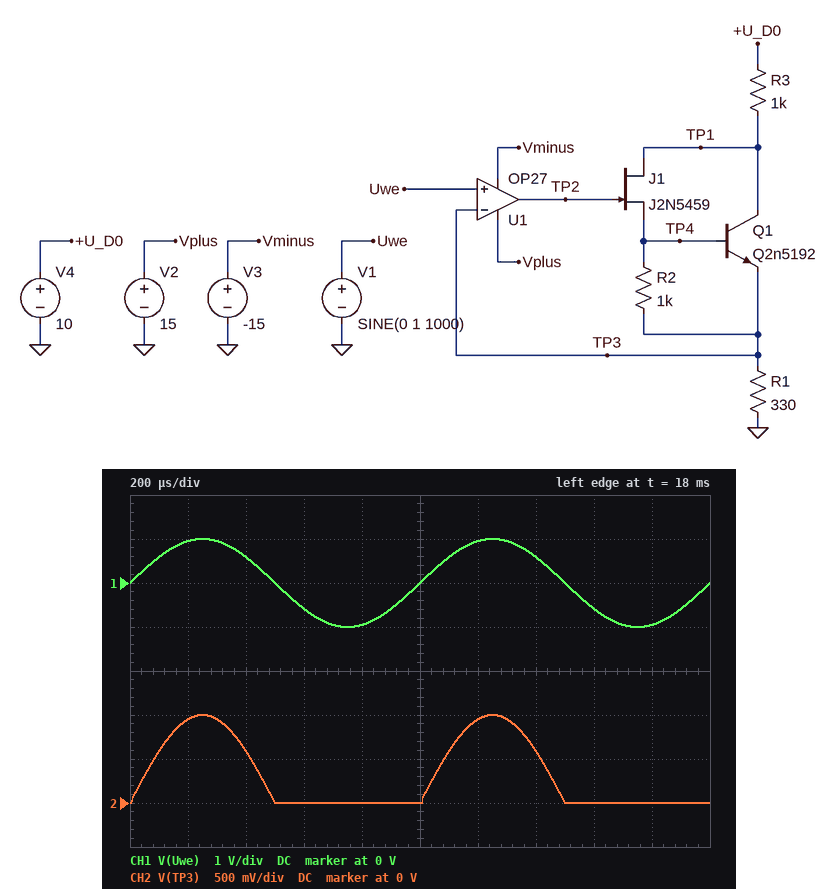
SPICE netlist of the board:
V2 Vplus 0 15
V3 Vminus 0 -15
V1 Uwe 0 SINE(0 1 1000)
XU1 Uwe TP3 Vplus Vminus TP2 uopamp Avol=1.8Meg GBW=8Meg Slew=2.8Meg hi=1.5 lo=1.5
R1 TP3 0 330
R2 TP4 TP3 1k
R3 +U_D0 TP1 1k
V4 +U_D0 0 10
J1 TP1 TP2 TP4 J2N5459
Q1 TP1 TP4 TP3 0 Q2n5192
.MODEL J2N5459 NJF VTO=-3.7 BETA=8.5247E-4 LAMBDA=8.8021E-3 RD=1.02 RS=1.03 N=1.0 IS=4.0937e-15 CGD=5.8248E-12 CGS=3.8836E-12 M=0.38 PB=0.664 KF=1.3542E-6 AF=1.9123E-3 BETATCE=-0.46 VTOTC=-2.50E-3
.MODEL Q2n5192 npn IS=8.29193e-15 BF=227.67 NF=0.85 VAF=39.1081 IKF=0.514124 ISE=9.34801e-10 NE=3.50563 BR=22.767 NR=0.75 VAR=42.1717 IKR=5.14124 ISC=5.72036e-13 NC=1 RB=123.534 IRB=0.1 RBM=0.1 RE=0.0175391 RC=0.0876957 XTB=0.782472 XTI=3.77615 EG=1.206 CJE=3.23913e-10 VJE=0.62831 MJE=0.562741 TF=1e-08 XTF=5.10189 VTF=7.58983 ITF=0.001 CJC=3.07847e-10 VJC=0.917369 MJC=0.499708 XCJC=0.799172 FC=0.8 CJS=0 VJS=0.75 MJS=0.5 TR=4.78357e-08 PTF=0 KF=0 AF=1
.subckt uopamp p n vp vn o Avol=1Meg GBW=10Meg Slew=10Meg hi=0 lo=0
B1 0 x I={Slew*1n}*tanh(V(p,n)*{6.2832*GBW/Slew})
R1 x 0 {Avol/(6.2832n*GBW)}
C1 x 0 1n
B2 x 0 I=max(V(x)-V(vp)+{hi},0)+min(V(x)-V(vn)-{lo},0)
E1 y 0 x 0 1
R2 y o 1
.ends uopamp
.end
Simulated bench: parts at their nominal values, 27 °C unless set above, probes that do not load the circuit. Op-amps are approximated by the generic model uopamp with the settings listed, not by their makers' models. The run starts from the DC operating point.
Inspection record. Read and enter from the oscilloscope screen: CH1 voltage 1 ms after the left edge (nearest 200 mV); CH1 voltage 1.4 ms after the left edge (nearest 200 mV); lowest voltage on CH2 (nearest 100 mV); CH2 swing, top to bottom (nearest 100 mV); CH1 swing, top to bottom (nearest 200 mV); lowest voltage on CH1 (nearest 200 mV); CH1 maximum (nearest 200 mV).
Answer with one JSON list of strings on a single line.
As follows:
["0 V", "600 mV", "0 V", "1.0 V", "2.0 V", "-1.0 V", "1.0 V"]
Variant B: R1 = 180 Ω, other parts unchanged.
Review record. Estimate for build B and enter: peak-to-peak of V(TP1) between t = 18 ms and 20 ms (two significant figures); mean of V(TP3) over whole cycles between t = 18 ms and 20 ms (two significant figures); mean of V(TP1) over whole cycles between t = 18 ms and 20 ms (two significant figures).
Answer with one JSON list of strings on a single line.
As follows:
["5.6 V", "320 mV", "8.2 V"]
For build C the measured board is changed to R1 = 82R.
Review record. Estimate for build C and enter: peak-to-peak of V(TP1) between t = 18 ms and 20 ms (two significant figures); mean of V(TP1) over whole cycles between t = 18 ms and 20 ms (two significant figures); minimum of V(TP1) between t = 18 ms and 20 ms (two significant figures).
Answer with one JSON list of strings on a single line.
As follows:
["8.6 V", "6.7 V", "1.4 V"]
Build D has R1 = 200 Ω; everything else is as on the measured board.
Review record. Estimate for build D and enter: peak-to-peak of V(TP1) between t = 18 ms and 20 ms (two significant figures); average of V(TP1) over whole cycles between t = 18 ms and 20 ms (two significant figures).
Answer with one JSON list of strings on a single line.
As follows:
["5.0 V", "8.4 V"]
